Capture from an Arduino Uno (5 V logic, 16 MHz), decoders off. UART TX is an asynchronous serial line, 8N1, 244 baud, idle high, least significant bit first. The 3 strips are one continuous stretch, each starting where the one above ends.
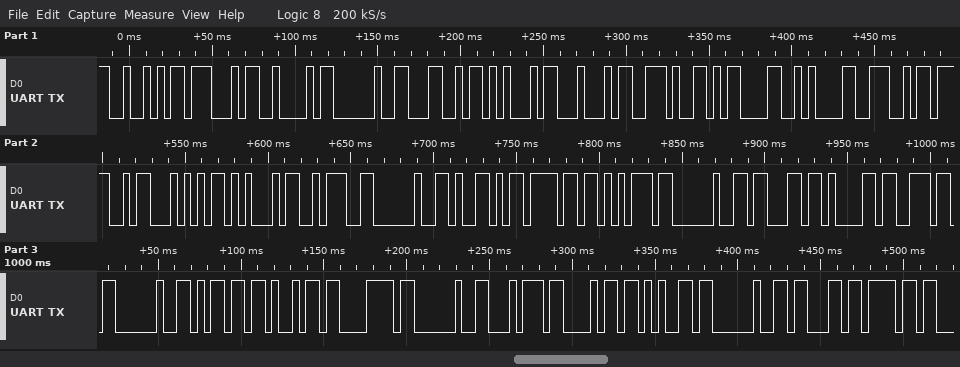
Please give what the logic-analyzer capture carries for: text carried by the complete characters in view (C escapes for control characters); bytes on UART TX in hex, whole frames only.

"RGB LED.\r\nNOTE: You can mix the co"
52 47 42 20 4C 45 44 2E 0D 0A 4E 4F 54 45 3A 20 59 6F 75 20 63 61 6E 20 6D 69 78 20 74 68 65 20 63 6F
